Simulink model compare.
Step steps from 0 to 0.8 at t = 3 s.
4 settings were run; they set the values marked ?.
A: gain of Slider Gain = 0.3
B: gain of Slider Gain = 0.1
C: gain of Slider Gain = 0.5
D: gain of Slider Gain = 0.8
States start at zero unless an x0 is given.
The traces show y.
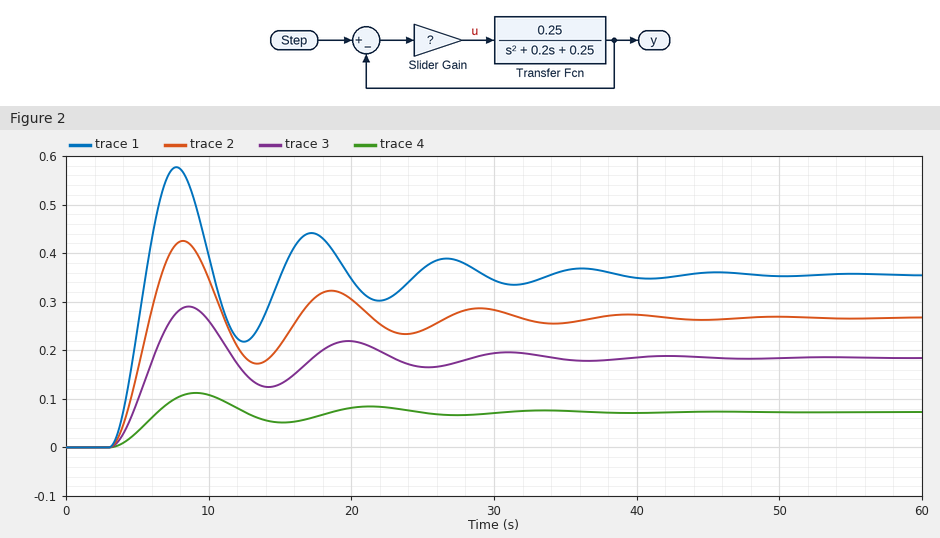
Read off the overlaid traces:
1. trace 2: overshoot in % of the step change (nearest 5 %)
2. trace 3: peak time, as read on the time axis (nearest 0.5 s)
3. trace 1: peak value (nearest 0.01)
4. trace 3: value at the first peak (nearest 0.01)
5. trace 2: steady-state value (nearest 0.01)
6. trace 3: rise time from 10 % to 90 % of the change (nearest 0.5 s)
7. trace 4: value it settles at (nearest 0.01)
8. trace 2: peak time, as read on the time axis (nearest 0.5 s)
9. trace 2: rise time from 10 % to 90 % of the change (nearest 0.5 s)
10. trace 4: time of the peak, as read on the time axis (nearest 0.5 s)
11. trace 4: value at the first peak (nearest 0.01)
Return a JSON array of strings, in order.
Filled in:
["60 %", "8.5 s", "0.58", "0.29", "0.27", "2.0 s", "0.07", "8.0 s", "2.0 s", "9.0 s", "0.11"]
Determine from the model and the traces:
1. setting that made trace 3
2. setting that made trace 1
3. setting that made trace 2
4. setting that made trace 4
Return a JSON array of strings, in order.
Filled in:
["A", "D", "C", "B"]
